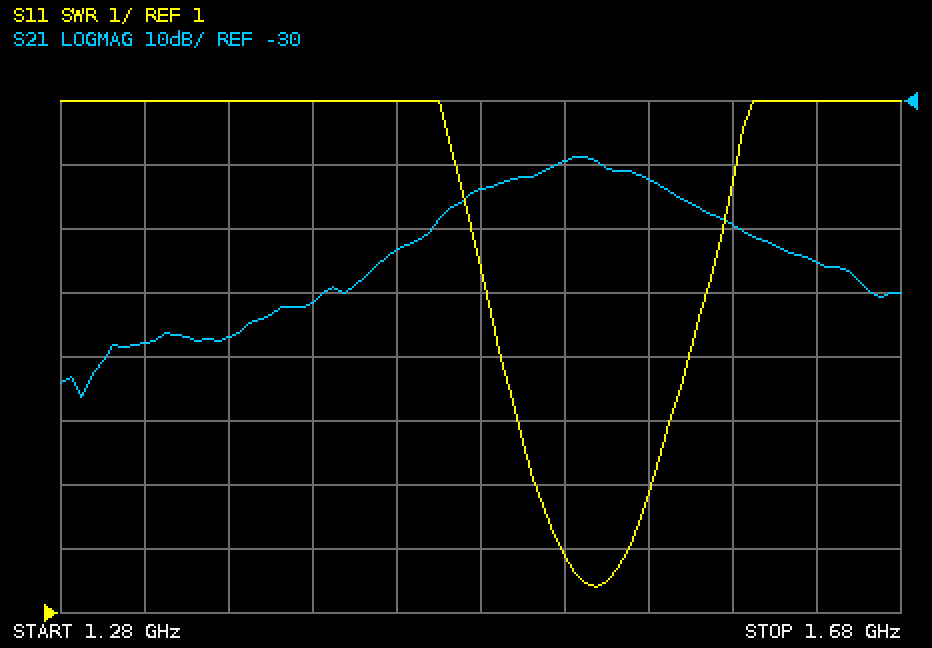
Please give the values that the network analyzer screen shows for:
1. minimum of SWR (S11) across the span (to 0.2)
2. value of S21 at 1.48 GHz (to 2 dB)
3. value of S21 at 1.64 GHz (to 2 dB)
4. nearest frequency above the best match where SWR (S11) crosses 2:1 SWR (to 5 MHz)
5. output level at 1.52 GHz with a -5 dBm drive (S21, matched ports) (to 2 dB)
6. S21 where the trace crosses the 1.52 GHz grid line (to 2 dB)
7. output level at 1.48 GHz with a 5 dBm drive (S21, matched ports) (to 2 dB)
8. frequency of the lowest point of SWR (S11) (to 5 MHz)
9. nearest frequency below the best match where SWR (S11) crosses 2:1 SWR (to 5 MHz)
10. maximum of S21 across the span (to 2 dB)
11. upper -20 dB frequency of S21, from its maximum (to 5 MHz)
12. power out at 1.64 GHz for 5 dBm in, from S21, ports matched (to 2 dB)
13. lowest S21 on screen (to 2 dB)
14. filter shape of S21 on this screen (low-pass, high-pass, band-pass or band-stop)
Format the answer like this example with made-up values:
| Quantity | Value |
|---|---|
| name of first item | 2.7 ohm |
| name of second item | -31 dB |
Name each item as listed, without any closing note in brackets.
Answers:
| Quantity | Value |
|---|---|
| minimum of SWR (S11) across the span | 1.4 |
| value of S21 at 1.48 GHz | -44 dB |
| value of S21 at 1.64 GHz | -56 dB |
| nearest frequency above the best match where SWR (S11) crosses 2:1 SWR | 1.550 GHz |
| output level at 1.52 GHz with a -5 dBm drive (S21, matched ports) | -44 dBm |
| S21 where the trace crosses the 1.52 GHz grid line | -40 dB |
| output level at 1.48 GHz with a 5 dBm drive (S21, matched ports) | -38 dBm |
| frequency of the lowest point of SWR (S11) | 1.535 GHz |
| nearest frequency below the best match where SWR (S11) crosses 2:1 SWR | 1.520 GHz |
| maximum of S21 across the span | -38 dB |
| upper -20 dB frequency of S21, from its maximum | 1.660 GHz |
| power out at 1.64 GHz for 5 dBm in, from S21, ports matched | -50 dBm |
| lowest S21 on screen | -76 dB |
| filter shape of S21 on this screen | band-pass |
